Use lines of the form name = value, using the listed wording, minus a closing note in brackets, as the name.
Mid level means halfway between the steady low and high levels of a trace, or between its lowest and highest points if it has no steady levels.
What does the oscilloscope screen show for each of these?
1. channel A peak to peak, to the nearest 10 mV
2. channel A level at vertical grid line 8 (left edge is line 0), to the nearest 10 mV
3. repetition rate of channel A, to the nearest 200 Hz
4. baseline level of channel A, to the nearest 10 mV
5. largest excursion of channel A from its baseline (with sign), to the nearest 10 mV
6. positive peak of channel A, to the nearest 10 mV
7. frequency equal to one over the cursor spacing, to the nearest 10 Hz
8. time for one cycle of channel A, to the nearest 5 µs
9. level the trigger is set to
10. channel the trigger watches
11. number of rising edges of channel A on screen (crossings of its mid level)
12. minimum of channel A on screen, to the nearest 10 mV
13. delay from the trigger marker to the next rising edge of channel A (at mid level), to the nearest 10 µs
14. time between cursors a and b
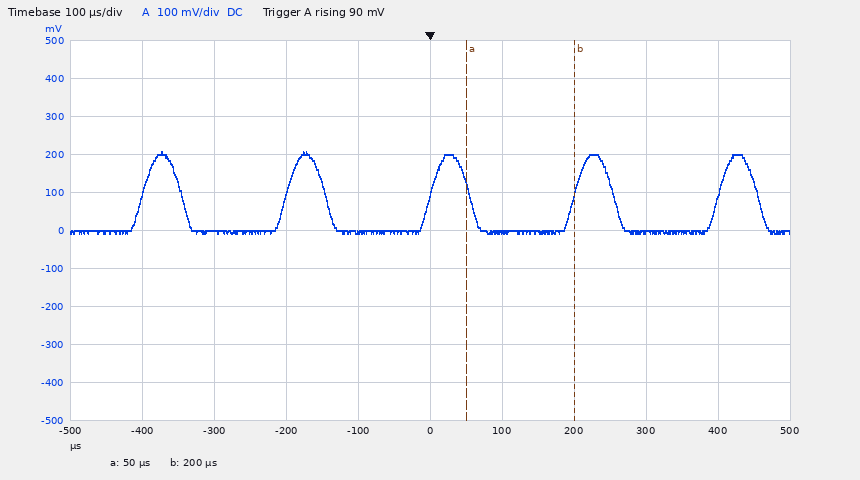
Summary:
channel A peak to peak, to the nearest 10 mV = 220 mV
channel A level at vertical grid line 8 (left edge is line 0), to the nearest 10 mV = 0 mV
repetition rate of channel A, to the nearest 200 Hz = 5.0 kHz
baseline level of channel A, to the nearest 10 mV = 0 mV
largest excursion of channel A from its baseline (with sign), to the nearest 10 mV = +210 mV
positive peak of channel A, to the nearest 10 mV = 210 mV
frequency equal to one over the cursor spacing, to the nearest 10 Hz = 6.67 kHz
time for one cycle of channel A, to the nearest 5 µs = 200 µs
level the trigger is set to = 90 mV
channel the trigger watches = channel A
number of rising edges of channel A on screen = 5
minimum of channel A on screen, to the nearest 10 mV = -10 mV
delay from the trigger marker to the next rising edge of channel A (at mid level), to the nearest 10 µs = 200 µs
time between cursors a and b = 150 µs
